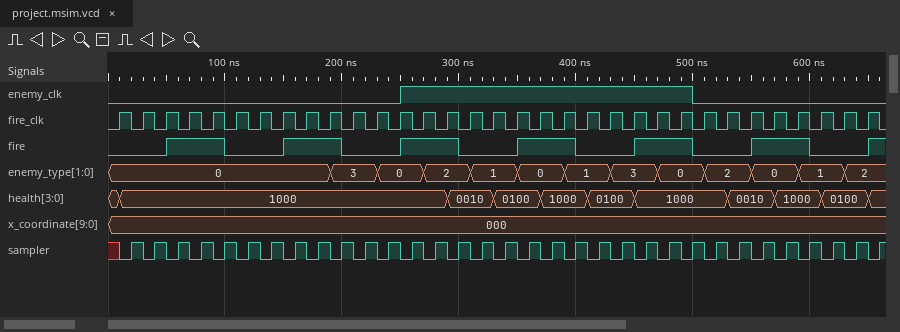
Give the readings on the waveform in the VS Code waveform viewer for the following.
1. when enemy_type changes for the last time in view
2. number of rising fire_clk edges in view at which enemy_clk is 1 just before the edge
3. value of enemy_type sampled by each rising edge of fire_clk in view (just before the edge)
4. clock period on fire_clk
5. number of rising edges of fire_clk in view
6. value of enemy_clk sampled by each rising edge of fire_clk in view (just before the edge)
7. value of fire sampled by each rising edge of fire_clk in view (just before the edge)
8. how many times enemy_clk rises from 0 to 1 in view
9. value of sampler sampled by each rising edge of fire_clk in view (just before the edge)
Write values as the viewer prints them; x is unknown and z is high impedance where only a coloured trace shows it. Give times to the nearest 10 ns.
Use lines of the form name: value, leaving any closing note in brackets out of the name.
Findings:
when enemy_type changes for the last time in view: 630 ns
number of rising fire_clk edges in view at which enemy_clk is 1 just before the edge: 12
value of enemy_type sampled by each rising edge of fire_clk in view: 0, 0, 0, 0, 0, 0, 0, 0, 0, 0, 3, 3, 0, 0, 2, 2, 1, 1, 0, 0, 1, 1, 3, 3, 0, 0, 2, 2, 0, 0, 1, 1, 2
clock period on fire_clk: 20 ns
number of rising edges of fire_clk in view: 33
value of enemy_clk sampled by each rising edge of fire_clk in view: 0 0 0 0 0 0 0 0 0 0 0 0 0 1 1 1 1 1 1 1 1 1 1 1 1 0 0 0 0 0 0 0 0
value of fire sampled by each rising edge of fire_clk in view: 0 0 0 1 1 0 0 0 1 1 0 0 0 1 1 0 0 0 1 1 0 0 0 1 1 0 0 0 1 1 0 0 0
how many times enemy_clk rises from 0 to 1 in view: 1
value of sampler sampled by each rising edge of fire_clk in view: x 1 1 1 1 1 1 1 1 1 1 1 1 1 1 1 1 1 1 1 1 1 1 1 1 1 1 1 1 1 1 1 1
